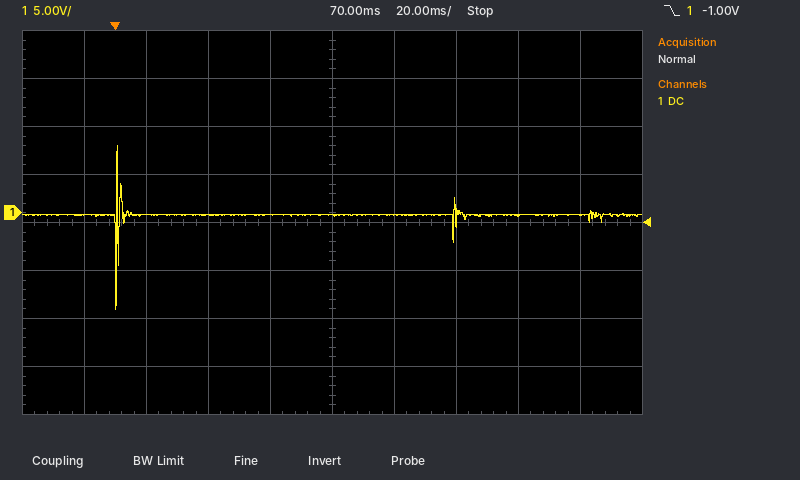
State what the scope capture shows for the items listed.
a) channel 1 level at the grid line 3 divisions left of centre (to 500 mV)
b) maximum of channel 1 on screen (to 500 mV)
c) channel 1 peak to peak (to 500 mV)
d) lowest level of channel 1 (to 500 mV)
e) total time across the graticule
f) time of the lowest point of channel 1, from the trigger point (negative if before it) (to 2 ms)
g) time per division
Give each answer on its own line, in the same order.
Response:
0.0 V
7.0 V
17.0 V
-10.0 V
200 ms
0 ms
20 ms
